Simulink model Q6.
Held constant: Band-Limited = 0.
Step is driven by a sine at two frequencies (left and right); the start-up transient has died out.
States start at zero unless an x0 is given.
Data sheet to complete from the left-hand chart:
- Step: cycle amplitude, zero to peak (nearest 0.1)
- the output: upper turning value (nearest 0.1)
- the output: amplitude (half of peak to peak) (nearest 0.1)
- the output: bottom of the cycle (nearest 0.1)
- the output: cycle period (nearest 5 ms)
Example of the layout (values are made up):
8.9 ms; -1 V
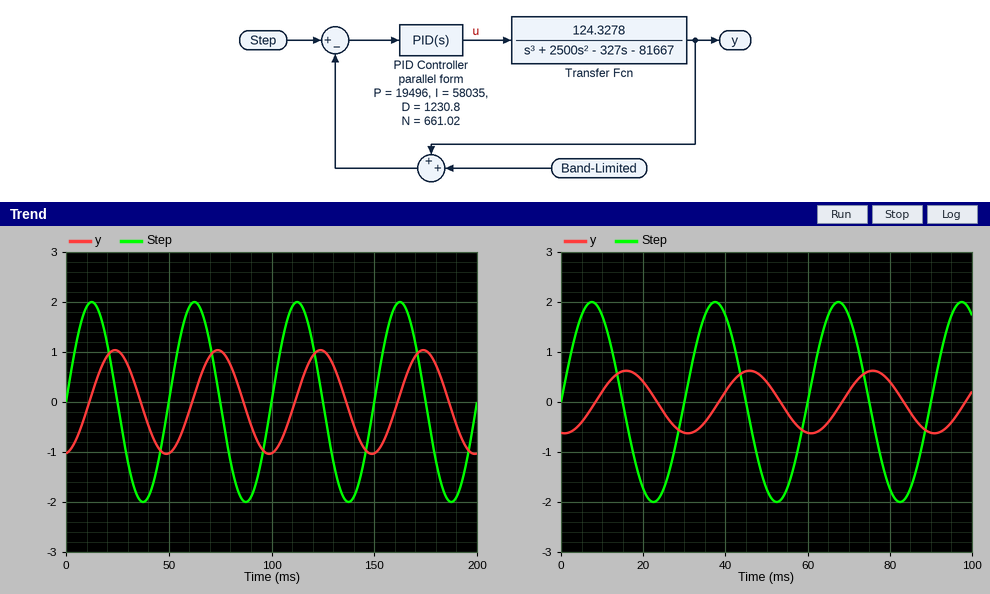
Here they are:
2.0; 1.0; 1.0; -1.0; 50 ms
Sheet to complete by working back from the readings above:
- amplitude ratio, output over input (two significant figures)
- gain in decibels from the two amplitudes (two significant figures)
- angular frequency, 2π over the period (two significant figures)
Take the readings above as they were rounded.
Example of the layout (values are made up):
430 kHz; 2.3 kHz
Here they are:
0.50; -6.0 dB; 0.13 rad/ms
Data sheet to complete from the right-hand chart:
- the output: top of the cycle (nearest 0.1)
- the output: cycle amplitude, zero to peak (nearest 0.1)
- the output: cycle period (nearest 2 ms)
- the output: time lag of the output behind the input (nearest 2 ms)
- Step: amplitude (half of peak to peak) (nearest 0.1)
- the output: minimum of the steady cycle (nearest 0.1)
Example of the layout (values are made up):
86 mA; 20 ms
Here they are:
0.6; 0.6; 30 ms; 8 ms; 2.0; -0.6
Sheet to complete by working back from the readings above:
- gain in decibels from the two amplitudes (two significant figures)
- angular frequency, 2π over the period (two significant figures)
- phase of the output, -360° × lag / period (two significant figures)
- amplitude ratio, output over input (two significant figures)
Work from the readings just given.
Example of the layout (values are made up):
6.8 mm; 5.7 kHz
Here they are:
-10 dB; 0.21 rad/ms; -96°; 0.30
